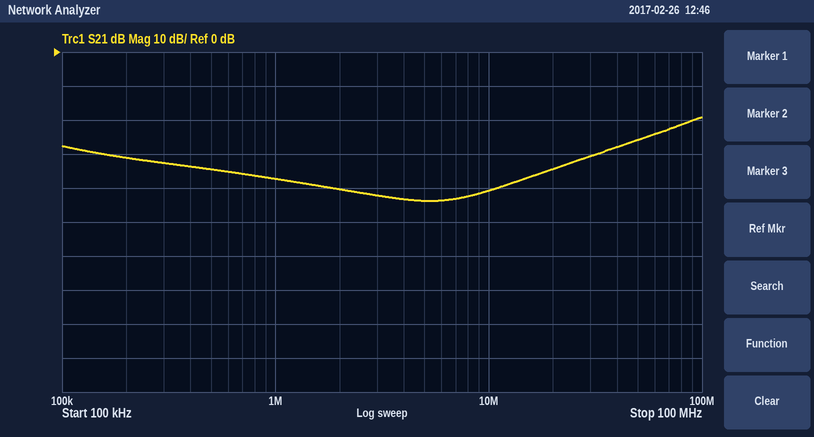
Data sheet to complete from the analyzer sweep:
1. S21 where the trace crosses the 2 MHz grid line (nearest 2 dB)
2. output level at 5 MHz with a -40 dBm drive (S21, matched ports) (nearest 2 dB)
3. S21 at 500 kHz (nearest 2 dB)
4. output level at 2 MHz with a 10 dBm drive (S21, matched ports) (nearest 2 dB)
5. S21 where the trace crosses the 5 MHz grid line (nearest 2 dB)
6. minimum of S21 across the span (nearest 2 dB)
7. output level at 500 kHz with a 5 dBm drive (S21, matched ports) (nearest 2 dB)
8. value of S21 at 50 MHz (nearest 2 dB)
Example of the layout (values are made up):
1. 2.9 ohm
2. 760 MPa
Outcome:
1. -40 dB
2. -84 dBm
3. -34 dB
4. -30 dBm
5. -44 dB
6. -44 dB
7. -30 dBm
8. -26 dB
